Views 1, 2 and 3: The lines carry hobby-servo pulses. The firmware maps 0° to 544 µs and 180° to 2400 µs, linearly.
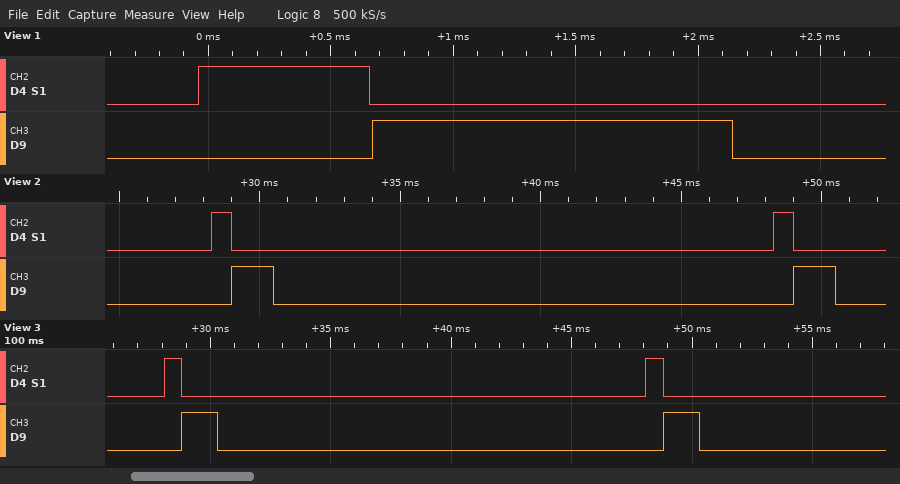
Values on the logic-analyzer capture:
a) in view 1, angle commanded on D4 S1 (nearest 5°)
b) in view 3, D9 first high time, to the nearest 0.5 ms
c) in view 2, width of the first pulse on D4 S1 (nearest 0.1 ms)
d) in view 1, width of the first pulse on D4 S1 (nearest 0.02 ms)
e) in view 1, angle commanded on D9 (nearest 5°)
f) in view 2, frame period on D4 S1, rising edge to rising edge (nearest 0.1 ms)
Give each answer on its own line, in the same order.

15°
1.5 ms
0.7 ms
0.70 ms
90°
20.0 ms
